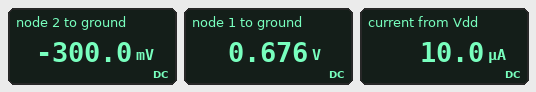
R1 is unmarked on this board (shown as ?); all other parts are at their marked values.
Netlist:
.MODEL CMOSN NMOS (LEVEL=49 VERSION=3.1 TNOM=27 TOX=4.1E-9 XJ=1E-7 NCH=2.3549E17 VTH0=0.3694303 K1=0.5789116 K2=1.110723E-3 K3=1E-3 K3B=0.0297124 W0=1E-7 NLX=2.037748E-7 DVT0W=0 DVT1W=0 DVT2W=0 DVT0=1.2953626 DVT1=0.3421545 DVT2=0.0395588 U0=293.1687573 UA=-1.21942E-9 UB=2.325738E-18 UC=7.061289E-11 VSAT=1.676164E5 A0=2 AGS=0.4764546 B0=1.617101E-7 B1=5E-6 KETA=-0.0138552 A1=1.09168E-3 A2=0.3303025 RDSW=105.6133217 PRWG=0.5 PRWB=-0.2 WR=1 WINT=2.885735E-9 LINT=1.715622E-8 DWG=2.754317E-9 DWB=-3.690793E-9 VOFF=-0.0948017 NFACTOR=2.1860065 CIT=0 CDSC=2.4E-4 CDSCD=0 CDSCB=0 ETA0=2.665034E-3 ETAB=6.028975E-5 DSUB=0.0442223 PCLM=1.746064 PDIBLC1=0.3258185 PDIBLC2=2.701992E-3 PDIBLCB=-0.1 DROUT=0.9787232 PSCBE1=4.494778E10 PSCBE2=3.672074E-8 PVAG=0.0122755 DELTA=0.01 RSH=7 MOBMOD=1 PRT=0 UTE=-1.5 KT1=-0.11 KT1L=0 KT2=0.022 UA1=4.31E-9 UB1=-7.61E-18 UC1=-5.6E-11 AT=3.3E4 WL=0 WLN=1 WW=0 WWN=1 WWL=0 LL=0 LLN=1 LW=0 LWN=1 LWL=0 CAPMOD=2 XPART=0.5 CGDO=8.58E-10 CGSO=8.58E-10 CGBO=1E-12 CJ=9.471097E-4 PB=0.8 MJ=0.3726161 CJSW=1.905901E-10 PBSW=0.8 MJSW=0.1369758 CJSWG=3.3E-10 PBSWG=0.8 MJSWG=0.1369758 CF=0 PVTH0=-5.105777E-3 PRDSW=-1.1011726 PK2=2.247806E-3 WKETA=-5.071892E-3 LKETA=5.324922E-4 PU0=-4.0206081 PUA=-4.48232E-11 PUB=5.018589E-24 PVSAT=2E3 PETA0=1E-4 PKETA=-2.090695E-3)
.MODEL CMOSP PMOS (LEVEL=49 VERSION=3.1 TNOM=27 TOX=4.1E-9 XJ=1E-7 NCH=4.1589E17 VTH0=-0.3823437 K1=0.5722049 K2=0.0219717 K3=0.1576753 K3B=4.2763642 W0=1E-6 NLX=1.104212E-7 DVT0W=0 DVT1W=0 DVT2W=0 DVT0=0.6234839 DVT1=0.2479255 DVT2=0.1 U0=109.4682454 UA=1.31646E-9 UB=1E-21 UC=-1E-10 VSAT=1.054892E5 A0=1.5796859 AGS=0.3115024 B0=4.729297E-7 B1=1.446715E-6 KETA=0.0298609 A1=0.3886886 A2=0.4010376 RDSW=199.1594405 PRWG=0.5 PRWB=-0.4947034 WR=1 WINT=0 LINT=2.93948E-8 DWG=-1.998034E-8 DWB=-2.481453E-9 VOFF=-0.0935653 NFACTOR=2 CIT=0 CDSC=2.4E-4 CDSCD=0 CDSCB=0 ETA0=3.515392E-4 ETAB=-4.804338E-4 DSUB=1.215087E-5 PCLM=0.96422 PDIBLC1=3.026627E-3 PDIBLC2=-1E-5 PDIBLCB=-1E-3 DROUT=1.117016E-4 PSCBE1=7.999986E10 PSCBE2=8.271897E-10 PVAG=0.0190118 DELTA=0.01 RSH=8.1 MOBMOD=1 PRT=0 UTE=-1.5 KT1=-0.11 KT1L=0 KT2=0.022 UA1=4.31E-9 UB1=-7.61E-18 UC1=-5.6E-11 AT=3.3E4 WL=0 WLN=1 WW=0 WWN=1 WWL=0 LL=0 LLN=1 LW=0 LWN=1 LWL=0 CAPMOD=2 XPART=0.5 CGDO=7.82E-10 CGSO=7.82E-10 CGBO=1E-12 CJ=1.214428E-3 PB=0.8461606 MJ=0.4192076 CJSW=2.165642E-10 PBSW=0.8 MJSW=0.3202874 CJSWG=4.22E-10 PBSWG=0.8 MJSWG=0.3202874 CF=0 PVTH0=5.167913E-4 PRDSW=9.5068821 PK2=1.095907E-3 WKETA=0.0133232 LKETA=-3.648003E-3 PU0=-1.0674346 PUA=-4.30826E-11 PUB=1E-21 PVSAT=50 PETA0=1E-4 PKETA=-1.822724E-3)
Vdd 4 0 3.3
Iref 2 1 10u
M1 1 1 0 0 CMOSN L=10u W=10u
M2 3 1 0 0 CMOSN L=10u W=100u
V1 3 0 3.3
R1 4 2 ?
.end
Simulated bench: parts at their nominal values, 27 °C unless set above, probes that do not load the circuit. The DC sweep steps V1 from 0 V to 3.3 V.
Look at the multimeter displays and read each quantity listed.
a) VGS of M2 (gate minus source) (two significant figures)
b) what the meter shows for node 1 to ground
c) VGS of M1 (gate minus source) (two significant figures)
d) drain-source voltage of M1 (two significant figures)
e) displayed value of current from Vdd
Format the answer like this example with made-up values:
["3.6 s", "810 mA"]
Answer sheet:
["680 mV", "0.676 V", "680 mV", "680 mV", "10.0 µA"]
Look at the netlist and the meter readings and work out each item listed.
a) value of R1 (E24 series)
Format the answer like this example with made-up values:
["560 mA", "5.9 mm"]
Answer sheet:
["360 kΩ"]
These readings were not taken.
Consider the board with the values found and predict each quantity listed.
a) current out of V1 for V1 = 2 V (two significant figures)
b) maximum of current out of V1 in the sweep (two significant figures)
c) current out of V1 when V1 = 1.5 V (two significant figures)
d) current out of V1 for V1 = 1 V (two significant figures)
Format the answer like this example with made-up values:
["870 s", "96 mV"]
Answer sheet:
["100 µA", "100 µA", "100 µA", "100 µA"]
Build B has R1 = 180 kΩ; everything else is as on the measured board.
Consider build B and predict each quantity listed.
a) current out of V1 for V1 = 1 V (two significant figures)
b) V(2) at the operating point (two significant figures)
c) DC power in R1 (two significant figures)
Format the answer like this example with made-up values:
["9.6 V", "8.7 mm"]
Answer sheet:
["100 µA", "1.5 V", "18 µW"]
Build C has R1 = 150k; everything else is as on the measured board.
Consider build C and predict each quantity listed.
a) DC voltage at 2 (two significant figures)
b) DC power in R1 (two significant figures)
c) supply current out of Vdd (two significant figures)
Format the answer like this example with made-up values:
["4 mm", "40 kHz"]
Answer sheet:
["1.8 V", "15 µW", "10 µA"]
